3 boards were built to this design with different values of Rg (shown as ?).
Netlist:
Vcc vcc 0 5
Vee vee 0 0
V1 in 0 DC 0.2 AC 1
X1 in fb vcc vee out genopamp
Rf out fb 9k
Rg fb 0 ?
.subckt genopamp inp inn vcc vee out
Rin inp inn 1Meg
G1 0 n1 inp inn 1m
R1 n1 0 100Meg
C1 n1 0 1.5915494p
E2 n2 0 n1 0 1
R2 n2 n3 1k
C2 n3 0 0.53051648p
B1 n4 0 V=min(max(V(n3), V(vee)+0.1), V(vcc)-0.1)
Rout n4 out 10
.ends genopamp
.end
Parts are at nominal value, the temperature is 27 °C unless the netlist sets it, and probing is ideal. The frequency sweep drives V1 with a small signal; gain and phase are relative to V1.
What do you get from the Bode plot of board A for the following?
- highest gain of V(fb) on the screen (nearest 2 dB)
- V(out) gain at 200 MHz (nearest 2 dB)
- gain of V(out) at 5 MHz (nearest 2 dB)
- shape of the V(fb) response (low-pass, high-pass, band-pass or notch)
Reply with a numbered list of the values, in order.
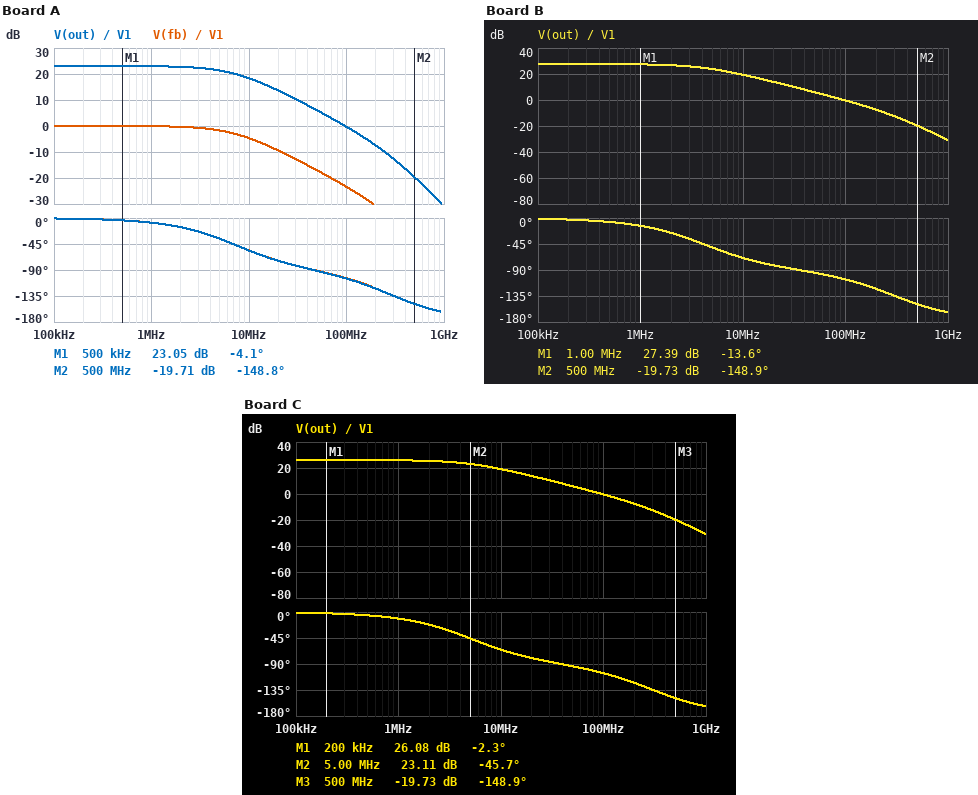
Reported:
1. 0 dB
2. -8 dB
3. 22 dB
4. low-pass
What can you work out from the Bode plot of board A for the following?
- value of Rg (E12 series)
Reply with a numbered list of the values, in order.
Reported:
1. 680 Ω
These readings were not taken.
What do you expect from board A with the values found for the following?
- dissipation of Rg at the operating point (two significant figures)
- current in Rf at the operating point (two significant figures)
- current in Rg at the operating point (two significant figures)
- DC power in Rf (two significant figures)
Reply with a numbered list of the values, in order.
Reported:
1. 59 µW
2. 290 µA
3. 290 µA
4. 780 µW
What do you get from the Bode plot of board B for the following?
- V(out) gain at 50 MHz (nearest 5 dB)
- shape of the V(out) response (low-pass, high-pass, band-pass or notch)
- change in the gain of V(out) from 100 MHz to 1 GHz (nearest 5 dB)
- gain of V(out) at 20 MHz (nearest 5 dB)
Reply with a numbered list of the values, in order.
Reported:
1. 5 dB
2. low-pass
3. -30 dB
4. 15 dB
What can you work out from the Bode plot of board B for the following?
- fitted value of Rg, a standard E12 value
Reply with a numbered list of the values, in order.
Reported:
1. 390 Ω
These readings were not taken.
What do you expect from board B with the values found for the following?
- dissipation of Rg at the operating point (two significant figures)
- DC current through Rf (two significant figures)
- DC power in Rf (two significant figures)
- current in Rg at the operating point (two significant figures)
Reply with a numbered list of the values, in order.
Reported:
1. 100 µW
2. 510 µA
3. 2.4 mW
4. 510 µA
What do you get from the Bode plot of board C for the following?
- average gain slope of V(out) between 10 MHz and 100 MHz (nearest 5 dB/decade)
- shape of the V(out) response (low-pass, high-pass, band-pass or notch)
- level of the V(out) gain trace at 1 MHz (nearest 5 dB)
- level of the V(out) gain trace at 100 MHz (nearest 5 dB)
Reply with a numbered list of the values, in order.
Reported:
1. -20 dB/decade
2. low-pass
3. 25 dB
4. 0 dB
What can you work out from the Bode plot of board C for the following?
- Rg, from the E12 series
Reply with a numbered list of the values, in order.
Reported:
1. 470 Ω
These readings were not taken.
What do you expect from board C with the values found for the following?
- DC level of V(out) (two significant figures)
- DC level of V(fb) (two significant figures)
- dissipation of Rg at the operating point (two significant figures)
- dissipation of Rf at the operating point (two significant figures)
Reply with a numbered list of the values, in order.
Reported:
1. 4.0 V
2. 200 mV
3. 85 µW
4. 1.6 mW
